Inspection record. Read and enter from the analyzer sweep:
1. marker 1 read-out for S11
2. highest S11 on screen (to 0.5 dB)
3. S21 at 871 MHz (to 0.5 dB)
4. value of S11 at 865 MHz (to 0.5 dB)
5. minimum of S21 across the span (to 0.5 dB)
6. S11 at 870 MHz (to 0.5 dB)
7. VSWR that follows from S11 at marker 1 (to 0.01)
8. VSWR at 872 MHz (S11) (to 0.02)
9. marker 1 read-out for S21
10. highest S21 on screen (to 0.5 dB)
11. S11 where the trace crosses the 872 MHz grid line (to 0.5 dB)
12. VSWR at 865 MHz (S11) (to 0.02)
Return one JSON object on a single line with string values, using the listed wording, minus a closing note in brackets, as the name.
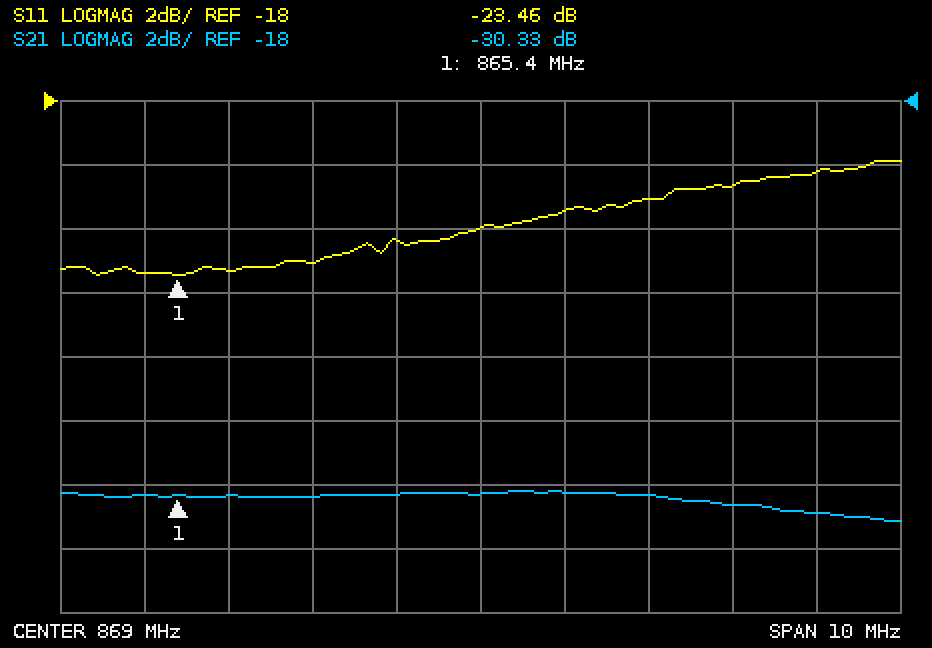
{"marker 1 read-out for S11": "-23.46 dB", "highest S11 on screen": "-20.0 dB", "S21 at 871 MHz": "-30.5 dB", "value of S11 at 865 MHz": "-23.5 dB", "minimum of S21 across the span": "-31.0 dB", "S11 at 870 MHz": "-21.5 dB", "VSWR that follows from S11 at marker 1": "1.14", "VSWR at 872 MHz (S11)": "1.20", "marker 1 read-out for S21": "-30.33 dB", "highest S21 on screen": "-30.0 dB", "S11 where the trace crosses the 872 MHz grid line": "-20.5 dB", "VSWR at 865 MHz (S11)": "1.14"}
